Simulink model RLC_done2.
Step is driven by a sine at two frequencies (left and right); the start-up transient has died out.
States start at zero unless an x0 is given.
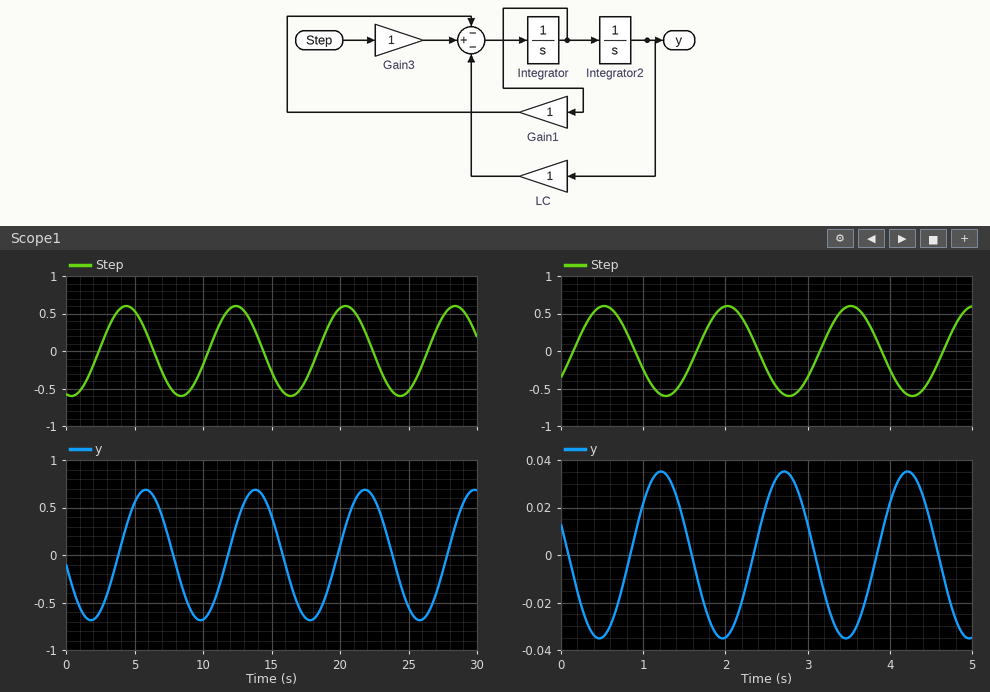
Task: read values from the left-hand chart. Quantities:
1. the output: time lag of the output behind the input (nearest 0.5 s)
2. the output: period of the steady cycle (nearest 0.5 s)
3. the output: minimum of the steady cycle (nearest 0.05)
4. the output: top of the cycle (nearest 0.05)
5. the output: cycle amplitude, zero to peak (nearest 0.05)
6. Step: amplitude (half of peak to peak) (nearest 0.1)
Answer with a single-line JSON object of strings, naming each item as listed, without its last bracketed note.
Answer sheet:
{"the output: time lag of the output behind the input": "1.5 s", "the output: period of the steady cycle": "8.0 s", "the output: minimum of the steady cycle": "-0.70", "the output: top of the cycle": "0.70", "the output: cycle amplitude, zero to peak": "0.70", "Step: amplitude (half of peak to peak)": "0.6"}
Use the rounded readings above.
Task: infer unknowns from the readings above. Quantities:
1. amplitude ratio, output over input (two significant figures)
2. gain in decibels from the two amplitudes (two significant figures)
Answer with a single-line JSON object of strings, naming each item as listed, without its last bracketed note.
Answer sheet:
{"amplitude ratio, output over input": "1.2", "gain in decibels from the two amplitudes": "1.3 dB"}
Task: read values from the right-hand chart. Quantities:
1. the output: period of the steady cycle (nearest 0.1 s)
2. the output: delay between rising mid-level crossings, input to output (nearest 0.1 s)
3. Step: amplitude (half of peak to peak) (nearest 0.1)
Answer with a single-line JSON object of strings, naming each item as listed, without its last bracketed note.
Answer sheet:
{"the output: period of the steady cycle": "1.5 s", "the output: delay between rising mid-level crossings, input to output": "0.7 s", "Step: amplitude (half of peak to peak)": "0.6"}
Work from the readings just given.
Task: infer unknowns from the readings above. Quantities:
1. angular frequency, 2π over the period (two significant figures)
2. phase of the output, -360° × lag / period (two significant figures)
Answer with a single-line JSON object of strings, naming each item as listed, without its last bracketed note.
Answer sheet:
{"angular frequency, 2π over the period": "4.2 rad/s", "phase of the output, -360° × lag / period": "-170°"}
